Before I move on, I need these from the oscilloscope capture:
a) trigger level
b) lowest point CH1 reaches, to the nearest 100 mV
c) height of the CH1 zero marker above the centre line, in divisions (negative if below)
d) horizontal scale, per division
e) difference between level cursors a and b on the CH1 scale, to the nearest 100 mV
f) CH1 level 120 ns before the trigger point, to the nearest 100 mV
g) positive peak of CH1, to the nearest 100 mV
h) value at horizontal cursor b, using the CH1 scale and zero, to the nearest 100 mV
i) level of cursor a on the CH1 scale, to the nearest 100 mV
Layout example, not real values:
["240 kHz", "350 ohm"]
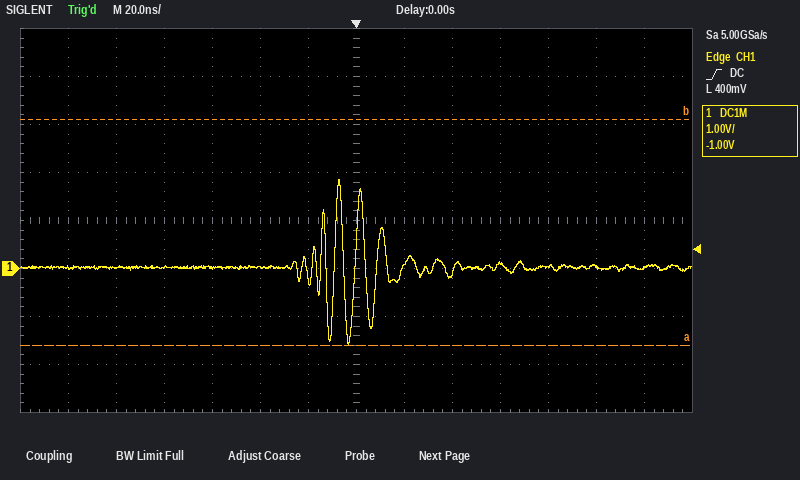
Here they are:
["400 mV", "-1.6 V", "-1.0 div", "20 ns", "4.7 V", "0.0 V", "1.9 V", "3.1 V", "-1.6 V"]
